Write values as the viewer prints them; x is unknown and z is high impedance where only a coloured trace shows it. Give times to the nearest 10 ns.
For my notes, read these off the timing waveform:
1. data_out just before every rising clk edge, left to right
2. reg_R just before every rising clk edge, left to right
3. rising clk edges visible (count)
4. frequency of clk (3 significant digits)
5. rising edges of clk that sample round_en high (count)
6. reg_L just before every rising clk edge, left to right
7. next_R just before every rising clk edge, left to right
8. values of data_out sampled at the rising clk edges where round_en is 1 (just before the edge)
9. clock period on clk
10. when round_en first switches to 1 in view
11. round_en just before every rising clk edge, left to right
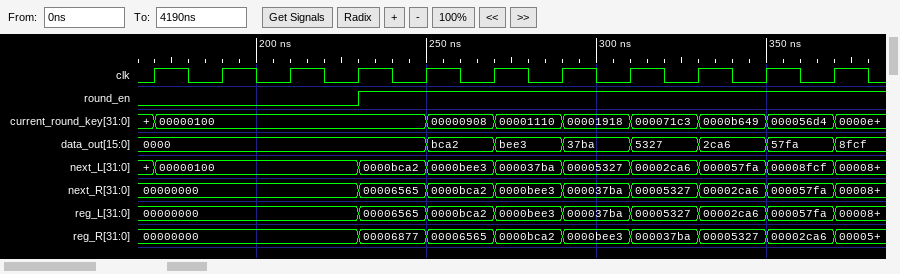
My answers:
0000, 0000, 0000, 0000, 0000, bca2, bee3, 37ba, 5327, 2ca6, 57fa
00000000, 00000000, 00000000, 00000000, 00006877, 00006565, 0000bca2, 0000bee3, 000037ba, 00005327, 00002ca6
11
50.0 MHz
7
00000000, 00000000, 00000000, 00000000, 00006565, 0000bca2, 0000bee3, 000037ba, 00005327, 00002ca6, 000057fa
00000000, 00000000, 00000000, 00000000, 00006565, 0000bca2, 0000bee3, 000037ba, 00005327, 00002ca6, 000057fa
0000, bca2, bee3, 37ba, 5327, 2ca6, 57fa
20 ns
230 ns
0 0 0 0 1 1 1 1 1 1 1
